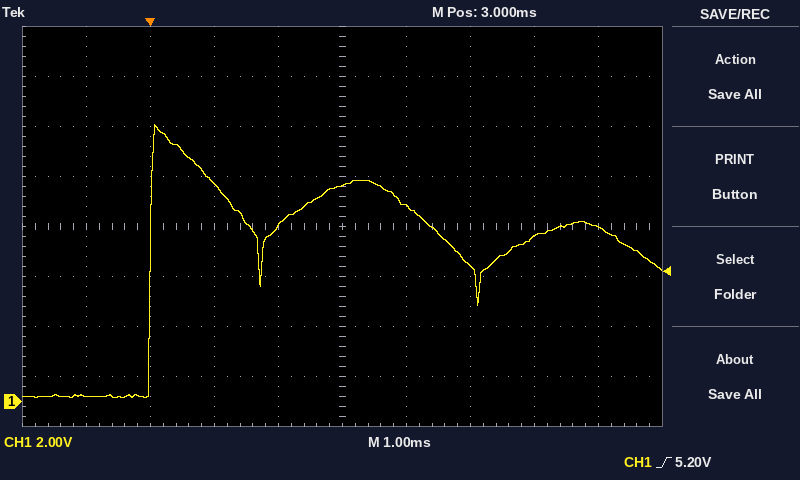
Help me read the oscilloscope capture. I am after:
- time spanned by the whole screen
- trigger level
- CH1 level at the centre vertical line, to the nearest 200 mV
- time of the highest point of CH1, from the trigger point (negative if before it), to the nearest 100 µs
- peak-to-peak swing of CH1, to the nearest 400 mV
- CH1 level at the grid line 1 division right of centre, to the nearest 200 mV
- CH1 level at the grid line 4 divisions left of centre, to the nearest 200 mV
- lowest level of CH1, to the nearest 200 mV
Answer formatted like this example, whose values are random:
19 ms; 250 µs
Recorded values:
10 ms; 5.20 V; 8.6 V; +100 µs; 10.8 V; 7.8 V; 200 mV; 200 mV
